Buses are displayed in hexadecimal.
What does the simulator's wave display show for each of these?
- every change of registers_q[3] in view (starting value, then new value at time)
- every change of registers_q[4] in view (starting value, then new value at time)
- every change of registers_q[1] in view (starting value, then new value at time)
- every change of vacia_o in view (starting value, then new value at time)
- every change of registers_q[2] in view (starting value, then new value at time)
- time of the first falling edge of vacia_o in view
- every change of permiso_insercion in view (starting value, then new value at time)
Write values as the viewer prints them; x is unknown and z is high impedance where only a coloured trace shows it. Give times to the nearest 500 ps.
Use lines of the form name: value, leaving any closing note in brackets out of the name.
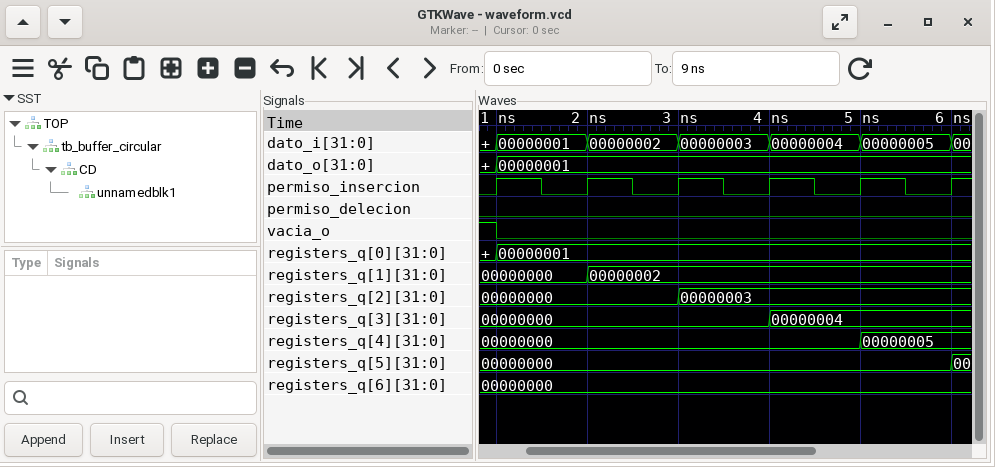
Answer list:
every change of registers_q[3] in view: 00000000, 00000004 at 4000 ps
every change of registers_q[4] in view: 00000000, 00000005 at 5000 ps
every change of registers_q[1] in view: 00000000, 00000002 at 2000 ps
every change of vacia_o in view: 1, 0 at 1000 ps
every change of registers_q[2] in view: 00000000, 00000003 at 3000 ps
time of the first falling edge of vacia_o in view: 1000 ps
every change of permiso_insercion in view: 0, 1 at 1000 ps, 0 at 1500 ps, 1 at 2000 ps, 0 at 2500 ps, 1 at 3000 ps, 0 at 3500 ps, 1 at 4000 ps, 0 at 4500 ps, 1 at 5000 ps, 0 at 5500 ps, 1 at 6000 ps
